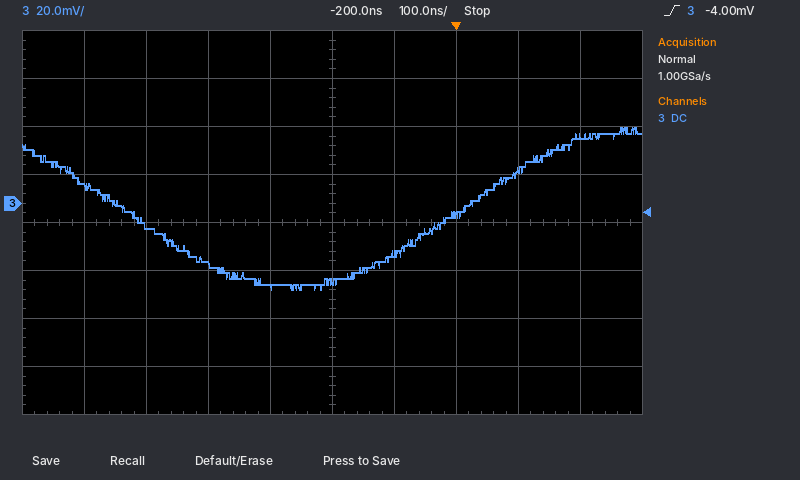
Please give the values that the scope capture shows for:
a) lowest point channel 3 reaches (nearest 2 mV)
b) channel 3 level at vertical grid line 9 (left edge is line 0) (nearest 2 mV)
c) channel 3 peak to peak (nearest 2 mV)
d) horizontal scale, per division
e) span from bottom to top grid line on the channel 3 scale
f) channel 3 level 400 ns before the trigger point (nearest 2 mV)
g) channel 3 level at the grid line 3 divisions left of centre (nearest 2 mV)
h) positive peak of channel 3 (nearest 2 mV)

-36 mV
28 mV
68 mV
100 ns
160 mV
-26 mV
-10 mV
32 mV
